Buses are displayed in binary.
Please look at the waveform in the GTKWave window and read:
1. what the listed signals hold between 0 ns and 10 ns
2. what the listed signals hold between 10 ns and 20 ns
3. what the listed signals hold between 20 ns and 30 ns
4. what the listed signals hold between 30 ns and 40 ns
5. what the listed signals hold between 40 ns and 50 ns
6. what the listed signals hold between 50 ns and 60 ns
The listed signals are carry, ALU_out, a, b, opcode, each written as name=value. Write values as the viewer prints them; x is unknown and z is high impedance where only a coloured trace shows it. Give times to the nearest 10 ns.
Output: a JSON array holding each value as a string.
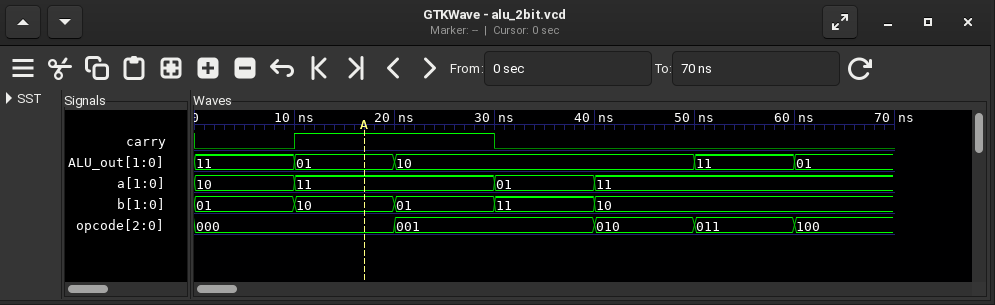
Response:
["carry=0, ALU_out=11, a=10, b=01, opcode=000", "carry=1, ALU_out=01, a=11, b=10, opcode=000", "carry=1, ALU_out=10, a=11, b=01, opcode=001", "carry=0, ALU_out=10, a=01, b=11, opcode=001", "carry=0, ALU_out=10, a=11, b=10, opcode=010", "carry=0, ALU_out=11, a=11, b=10, opcode=011"]
